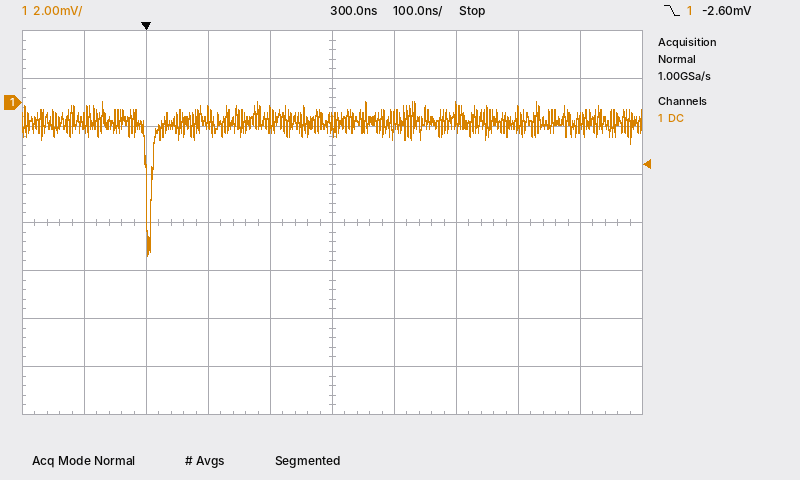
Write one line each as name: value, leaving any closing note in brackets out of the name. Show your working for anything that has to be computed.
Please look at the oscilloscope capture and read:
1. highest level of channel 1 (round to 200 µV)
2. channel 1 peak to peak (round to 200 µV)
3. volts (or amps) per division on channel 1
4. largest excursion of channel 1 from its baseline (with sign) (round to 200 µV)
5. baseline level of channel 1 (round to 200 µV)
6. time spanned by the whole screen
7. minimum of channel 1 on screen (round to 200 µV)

highest level of channel 1: 0.0 mV
channel 1 peak to peak: 0.0 mV − (-6.4 mV) = 6.4 mV
volts (or amps) per division on channel 1: 2 mV
largest excursion of channel 1 from its baseline (with sign): -6.4 mV − (-800 µV) = -5.6 mV
baseline level of channel 1: -800 µV
time spanned by the whole screen: 1 µs
minimum of channel 1 on screen: -6.4 mV
